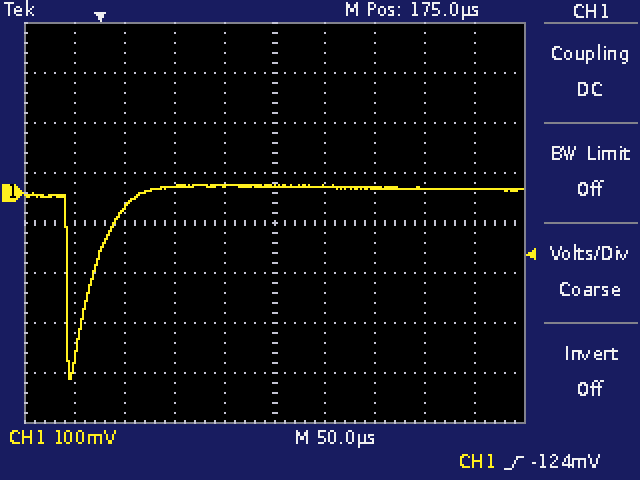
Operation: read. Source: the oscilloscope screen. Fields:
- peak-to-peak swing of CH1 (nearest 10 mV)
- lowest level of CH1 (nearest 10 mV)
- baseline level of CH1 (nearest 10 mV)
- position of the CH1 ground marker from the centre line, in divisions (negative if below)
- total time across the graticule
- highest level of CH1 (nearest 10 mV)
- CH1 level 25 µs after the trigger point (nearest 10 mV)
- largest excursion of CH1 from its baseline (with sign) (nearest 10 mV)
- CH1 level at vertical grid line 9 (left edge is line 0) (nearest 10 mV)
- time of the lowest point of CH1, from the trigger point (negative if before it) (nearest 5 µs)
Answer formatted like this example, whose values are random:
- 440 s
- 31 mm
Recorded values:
- 390 mV
- -370 mV
- 10 mV
- +0.6 div
- 500 µs
- 20 mV
- -30 mV
- -380 mV
- 10 mV
- -30 µs
